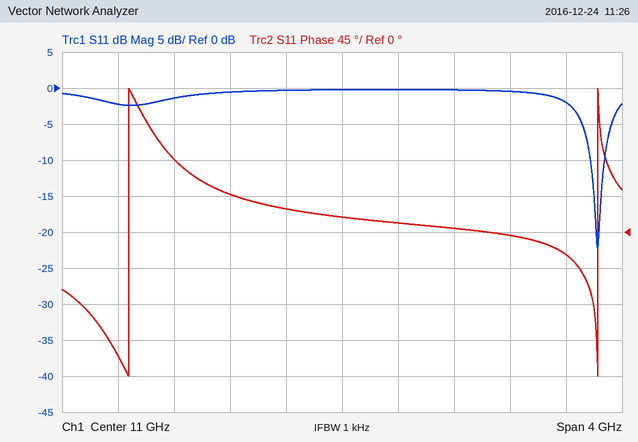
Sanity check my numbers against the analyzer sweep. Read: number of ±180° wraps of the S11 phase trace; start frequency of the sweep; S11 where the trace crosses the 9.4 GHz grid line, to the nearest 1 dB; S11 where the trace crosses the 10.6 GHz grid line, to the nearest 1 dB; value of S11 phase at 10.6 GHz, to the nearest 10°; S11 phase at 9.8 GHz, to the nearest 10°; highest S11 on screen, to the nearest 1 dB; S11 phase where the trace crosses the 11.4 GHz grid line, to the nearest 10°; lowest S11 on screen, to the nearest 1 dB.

2
9 GHz
-2 dB
0 dB
30°
90°
0 dB
10°
-22 dB
